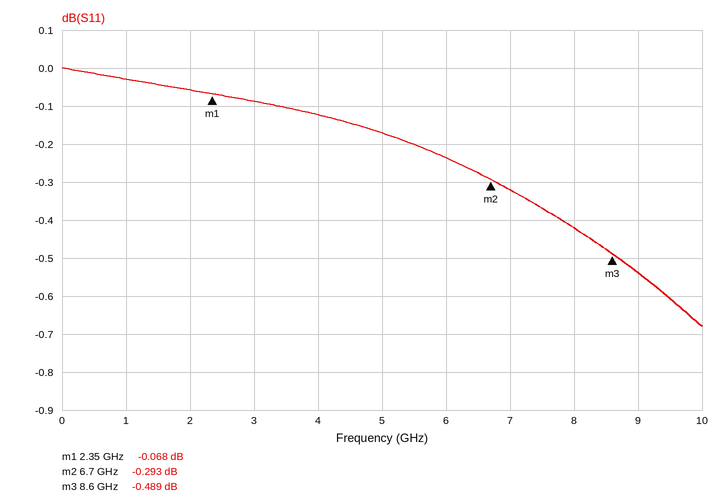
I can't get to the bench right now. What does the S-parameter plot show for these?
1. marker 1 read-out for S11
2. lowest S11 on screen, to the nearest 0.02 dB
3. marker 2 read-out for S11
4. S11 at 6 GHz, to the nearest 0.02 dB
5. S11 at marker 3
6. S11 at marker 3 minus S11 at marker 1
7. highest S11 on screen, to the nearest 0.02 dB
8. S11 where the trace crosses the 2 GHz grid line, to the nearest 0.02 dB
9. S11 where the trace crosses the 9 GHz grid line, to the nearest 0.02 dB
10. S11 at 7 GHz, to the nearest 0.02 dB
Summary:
-0.068 dB
-0.68 dB
-0.293 dB
-0.24 dB
-0.489 dB
-0.421 dB
0.00 dB
-0.06 dB
-0.54 dB
-0.32 dB
